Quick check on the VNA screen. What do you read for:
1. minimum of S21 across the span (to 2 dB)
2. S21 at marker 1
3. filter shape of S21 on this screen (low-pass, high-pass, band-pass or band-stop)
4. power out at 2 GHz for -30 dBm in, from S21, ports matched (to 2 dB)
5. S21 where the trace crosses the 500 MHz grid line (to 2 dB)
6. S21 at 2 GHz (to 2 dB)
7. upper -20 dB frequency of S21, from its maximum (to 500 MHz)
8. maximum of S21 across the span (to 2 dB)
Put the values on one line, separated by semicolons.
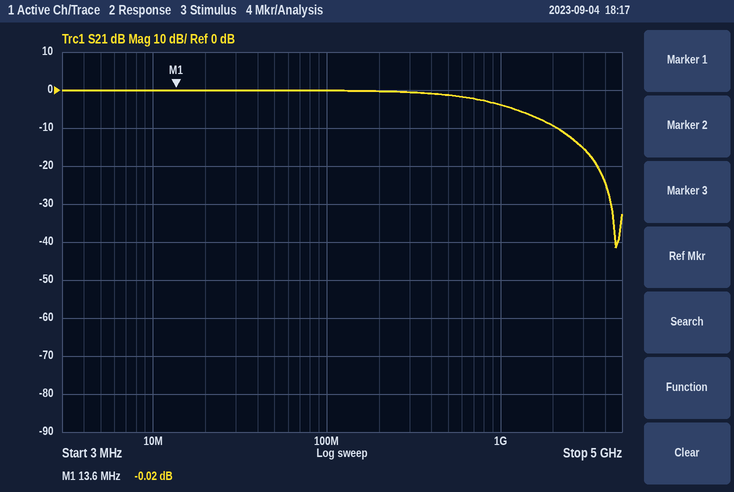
-42 dB; -0.02 dB; low-pass; -40 dBm; -2 dB; -10 dB; 3.5 GHz; 0 dB
